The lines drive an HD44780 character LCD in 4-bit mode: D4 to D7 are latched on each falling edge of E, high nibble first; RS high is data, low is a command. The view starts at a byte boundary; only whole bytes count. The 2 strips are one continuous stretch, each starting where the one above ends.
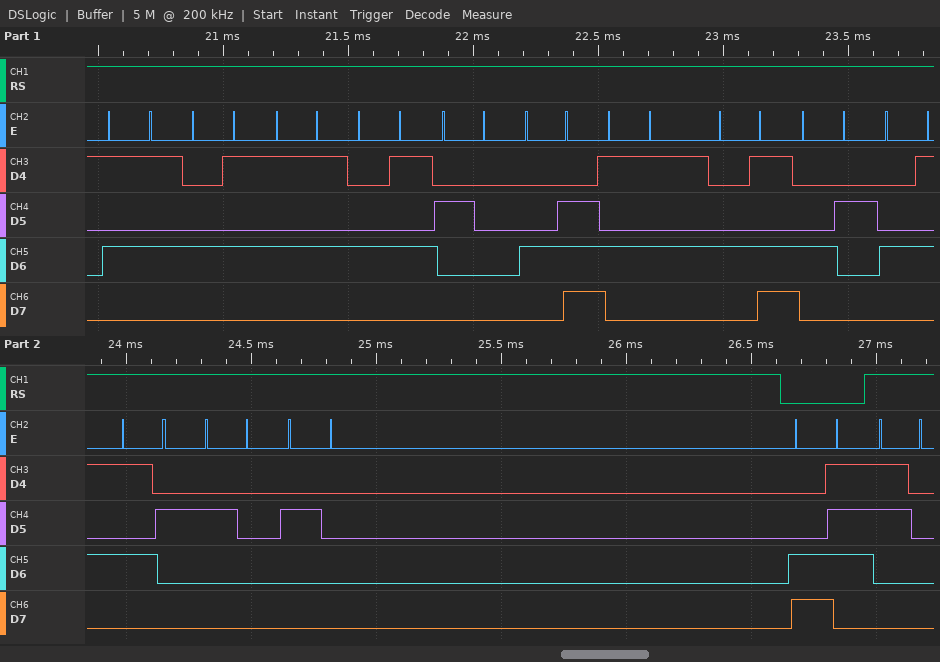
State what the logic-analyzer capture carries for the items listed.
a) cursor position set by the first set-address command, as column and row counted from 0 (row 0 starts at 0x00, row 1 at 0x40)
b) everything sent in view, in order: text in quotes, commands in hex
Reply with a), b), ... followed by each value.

a) column 7, row 1
b) "UEUE NUMBER  " 0xC7 "0"
